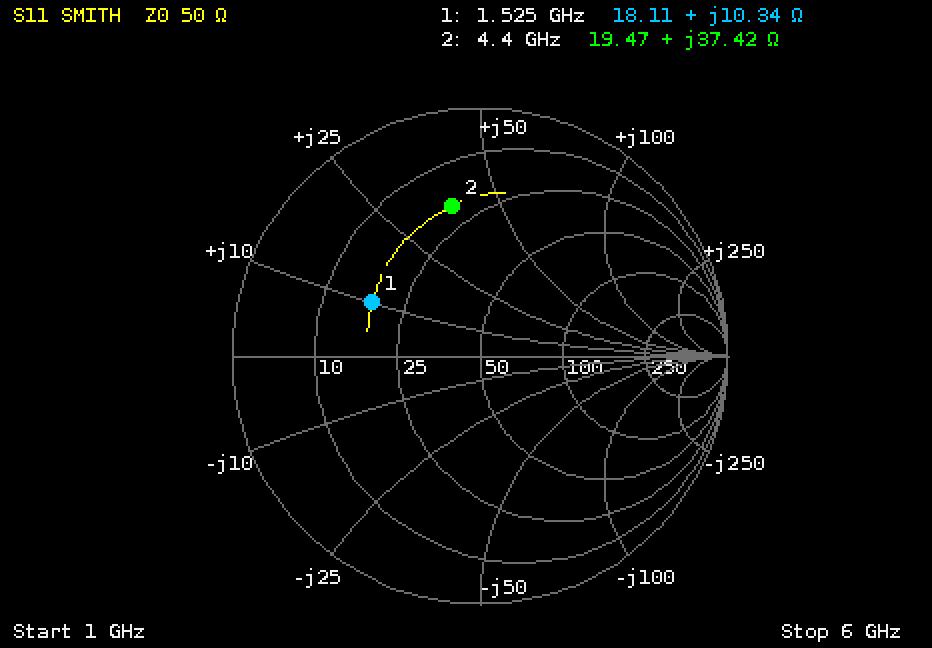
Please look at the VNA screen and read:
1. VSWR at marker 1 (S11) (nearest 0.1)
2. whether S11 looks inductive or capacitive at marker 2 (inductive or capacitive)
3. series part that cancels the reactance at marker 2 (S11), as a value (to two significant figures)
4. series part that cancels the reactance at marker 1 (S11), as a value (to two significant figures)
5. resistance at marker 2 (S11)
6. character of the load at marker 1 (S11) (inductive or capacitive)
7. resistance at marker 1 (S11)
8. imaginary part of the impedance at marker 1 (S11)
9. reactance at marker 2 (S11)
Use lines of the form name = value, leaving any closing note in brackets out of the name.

VSWR at marker 1 (S11) = 2.9
whether S11 looks inductive or capacitive at marker 2 = inductive
series part that cancels the reactance at marker 2 (S11), as a value = 970 fF
series part that cancels the reactance at marker 1 (S11), as a value = 10 pF
resistance at marker 2 = 19.47 Ω
character of the load at marker 1 (S11) = inductive
resistance at marker 1 = 18.11 Ω
imaginary part of the impedance at marker 1 = +10.34 Ω
reactance at marker 2 = +37.42 Ω
